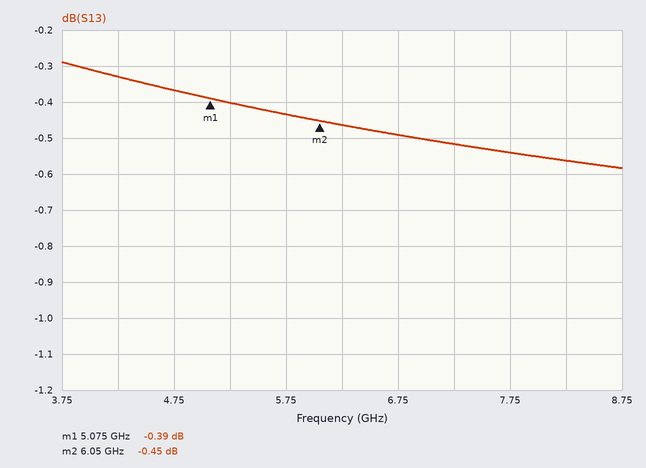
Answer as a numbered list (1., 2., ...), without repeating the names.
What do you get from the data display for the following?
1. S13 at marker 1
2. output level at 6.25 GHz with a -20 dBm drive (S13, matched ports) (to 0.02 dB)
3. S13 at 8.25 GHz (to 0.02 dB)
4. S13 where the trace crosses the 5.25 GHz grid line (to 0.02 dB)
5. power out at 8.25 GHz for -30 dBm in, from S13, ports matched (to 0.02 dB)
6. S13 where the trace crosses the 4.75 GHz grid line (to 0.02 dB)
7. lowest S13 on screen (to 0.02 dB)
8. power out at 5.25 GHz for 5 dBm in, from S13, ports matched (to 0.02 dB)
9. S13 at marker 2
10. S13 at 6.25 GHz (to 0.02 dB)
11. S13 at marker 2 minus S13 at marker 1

1. -0.39 dB
2. -20.46 dBm
3. -0.56 dB
4. -0.40 dB
5. -30.56 dBm
6. -0.36 dB
7. -0.58 dB
8. 4.60 dBm
9. -0.45 dB
10. -0.46 dB
11. -0.06 dB
